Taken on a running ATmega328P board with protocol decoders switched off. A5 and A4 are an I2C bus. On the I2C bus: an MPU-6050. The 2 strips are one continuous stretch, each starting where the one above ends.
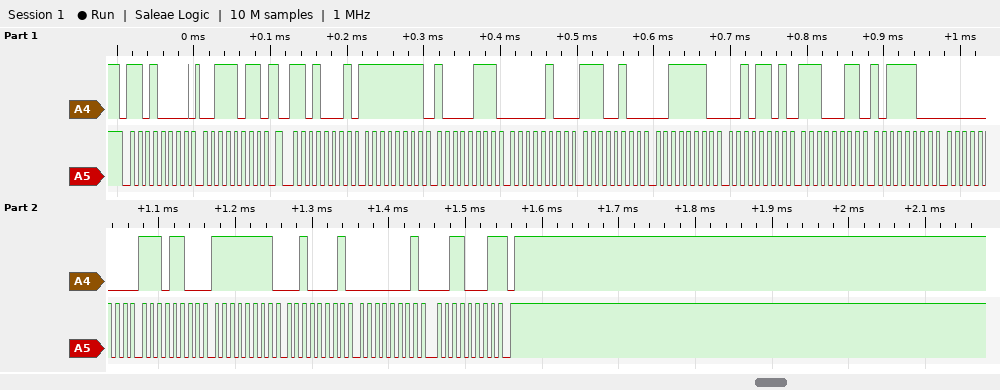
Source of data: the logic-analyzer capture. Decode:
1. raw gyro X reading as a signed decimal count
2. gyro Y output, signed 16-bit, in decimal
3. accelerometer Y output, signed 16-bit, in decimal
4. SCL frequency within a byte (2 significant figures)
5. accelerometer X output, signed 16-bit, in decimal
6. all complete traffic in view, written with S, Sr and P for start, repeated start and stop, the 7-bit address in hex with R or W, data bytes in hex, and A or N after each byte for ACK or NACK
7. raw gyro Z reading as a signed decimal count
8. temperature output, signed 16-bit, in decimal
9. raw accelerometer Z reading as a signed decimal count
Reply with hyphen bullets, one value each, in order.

- 236
- -223
- 1252
- 100 kHz
- -121
- S 68W A 3B A Sr 68R A FF A 87 A 04 A E4 A 3E A 2D A E3 A BC A 00 A EC A FF A 21 A 01 A 31 N P
- 305
- -7236
- 15917
